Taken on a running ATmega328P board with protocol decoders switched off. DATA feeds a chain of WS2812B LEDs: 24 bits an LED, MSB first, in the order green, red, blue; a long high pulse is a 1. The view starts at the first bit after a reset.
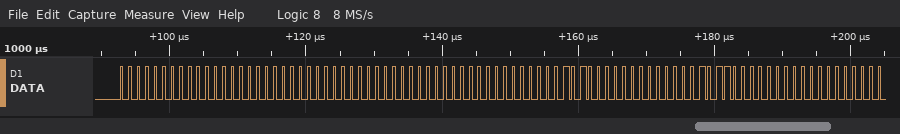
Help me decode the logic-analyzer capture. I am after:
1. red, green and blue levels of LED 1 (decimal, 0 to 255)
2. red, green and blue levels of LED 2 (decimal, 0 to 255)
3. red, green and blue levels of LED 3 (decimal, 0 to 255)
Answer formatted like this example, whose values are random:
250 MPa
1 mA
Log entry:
0, 0, 0
0, 0, 0
0, 10, 11
